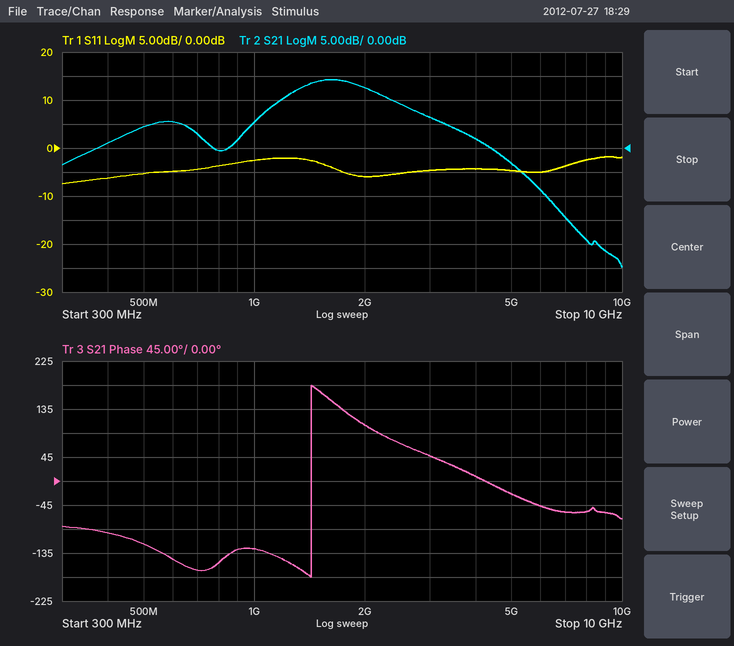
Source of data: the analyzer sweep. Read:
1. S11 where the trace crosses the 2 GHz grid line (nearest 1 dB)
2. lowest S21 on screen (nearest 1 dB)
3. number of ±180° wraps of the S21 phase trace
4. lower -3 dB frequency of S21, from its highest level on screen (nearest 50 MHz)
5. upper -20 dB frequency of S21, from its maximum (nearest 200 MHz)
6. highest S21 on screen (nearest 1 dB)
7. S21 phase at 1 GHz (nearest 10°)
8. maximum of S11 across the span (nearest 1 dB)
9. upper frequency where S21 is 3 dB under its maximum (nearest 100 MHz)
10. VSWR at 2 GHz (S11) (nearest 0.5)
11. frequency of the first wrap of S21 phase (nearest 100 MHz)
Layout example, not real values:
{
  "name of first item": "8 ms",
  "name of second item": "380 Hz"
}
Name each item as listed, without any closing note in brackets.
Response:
{
  "S11 where the trace crosses the 2 GHz grid line": "-6 dB",
  "lowest S21 on screen": "-25 dB",
  "number of ±180° wraps of the S21 phase trace": "1",
  "lower -3 dB frequency of S21, from its highest level on screen": "1.25 GHz",
  "upper -20 dB frequency of S21, from its maximum": "5.4 GHz",
  "highest S21 on screen": "14 dB",
  "S21 phase at 1 GHz": "-130°",
  "maximum of S11 across the span": "-2 dB",
  "upper frequency where S21 is 3 dB under its maximum": "2.2 GHz",
  "VSWR at 2 GHz (S11)": "3.0",
  "frequency of the first wrap of S21 phase": "1.4 GHz"
}
